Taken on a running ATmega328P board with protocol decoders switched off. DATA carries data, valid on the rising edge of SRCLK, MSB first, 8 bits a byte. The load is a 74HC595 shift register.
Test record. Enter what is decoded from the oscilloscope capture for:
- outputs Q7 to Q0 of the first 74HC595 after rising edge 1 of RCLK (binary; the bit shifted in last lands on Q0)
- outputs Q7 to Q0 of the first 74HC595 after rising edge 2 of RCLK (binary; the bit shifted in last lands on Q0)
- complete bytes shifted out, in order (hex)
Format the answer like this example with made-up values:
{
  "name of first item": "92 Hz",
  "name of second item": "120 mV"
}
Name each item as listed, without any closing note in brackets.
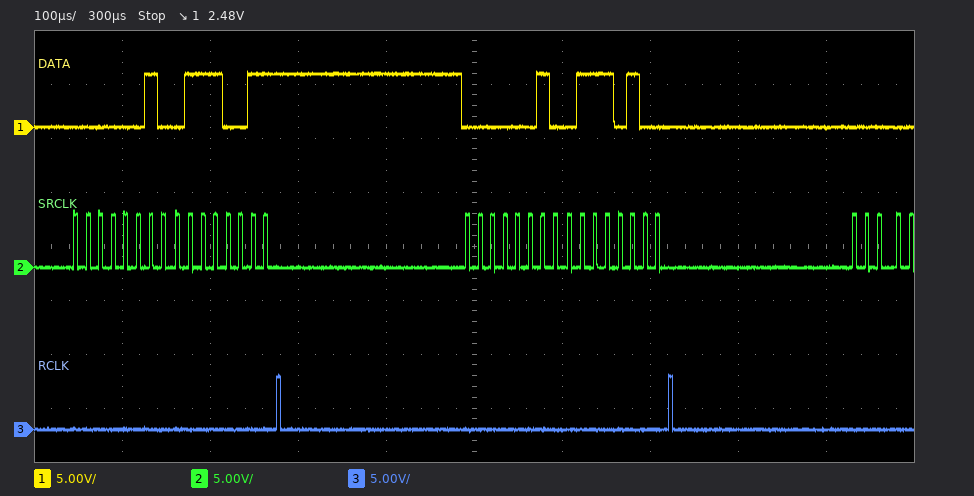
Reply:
{
  "outputs Q7 to Q0 of the first 74HC595 after rising edge 1 of RCLK": "01110011",
  "outputs Q7 to Q0 of the first 74HC595 after rising edge 2 of RCLK": "01110100",
  "complete bytes shifted out, in order": "02 73 02 74"
}
